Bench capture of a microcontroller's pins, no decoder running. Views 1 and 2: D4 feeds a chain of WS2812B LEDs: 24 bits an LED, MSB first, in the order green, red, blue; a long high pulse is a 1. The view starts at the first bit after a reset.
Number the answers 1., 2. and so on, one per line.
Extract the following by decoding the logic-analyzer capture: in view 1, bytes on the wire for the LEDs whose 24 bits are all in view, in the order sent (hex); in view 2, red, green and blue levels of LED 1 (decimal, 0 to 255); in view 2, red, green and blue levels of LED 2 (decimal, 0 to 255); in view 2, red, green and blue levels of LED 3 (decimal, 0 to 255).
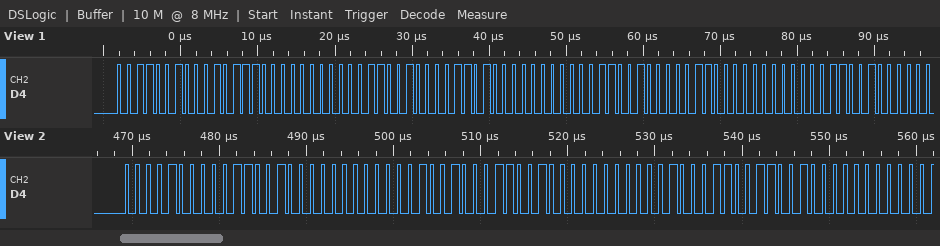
1. 32 2E 00 32 1A 00 32 0C 00
2. 50, 8, 0
3. 50, 18, 0
4. 50, 35, 0
